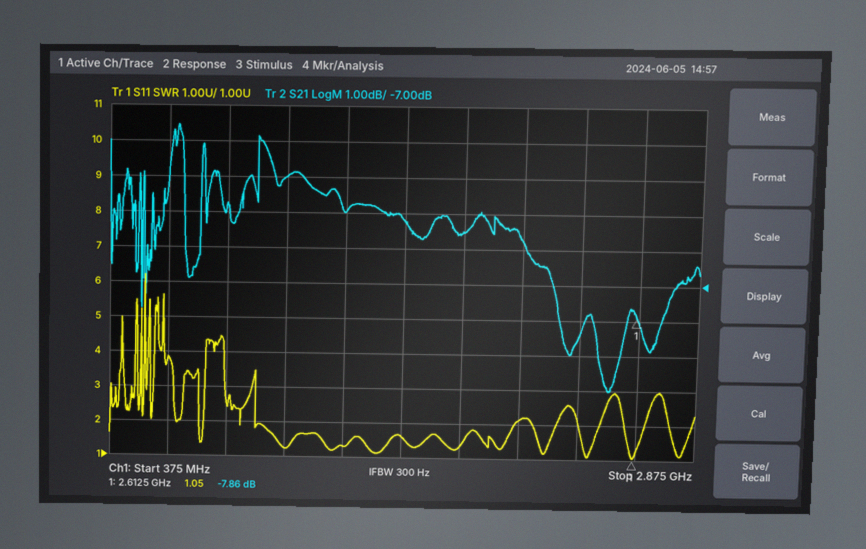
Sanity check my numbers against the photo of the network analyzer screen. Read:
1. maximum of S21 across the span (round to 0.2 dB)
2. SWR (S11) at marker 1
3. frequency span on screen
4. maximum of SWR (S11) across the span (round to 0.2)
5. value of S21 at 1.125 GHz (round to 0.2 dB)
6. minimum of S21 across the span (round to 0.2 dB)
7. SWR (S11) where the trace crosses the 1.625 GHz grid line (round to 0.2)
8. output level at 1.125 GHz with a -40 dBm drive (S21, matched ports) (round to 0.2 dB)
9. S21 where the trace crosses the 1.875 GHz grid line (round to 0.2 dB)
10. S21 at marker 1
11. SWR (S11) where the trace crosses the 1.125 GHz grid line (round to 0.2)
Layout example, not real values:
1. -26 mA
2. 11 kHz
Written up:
1. -2.6 dB
2. 1.05
3. 2.5 GHz
4. 6.2
5. -4.0 dB
6. -10.0 dB
7. 1.6
8. -44.0 dBm
9. -5.6 dB
10. -7.86 dB
11. 1.2
